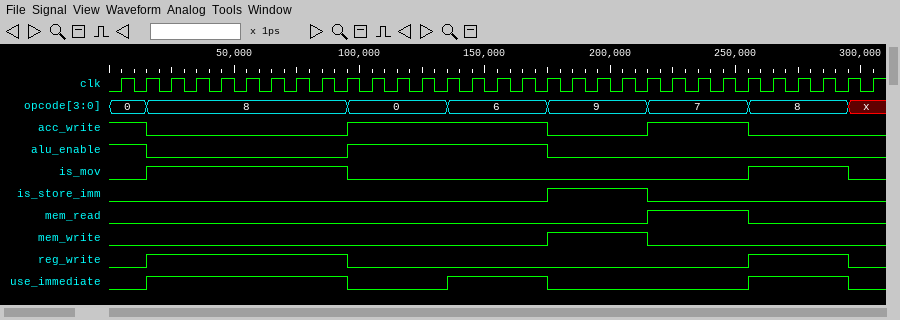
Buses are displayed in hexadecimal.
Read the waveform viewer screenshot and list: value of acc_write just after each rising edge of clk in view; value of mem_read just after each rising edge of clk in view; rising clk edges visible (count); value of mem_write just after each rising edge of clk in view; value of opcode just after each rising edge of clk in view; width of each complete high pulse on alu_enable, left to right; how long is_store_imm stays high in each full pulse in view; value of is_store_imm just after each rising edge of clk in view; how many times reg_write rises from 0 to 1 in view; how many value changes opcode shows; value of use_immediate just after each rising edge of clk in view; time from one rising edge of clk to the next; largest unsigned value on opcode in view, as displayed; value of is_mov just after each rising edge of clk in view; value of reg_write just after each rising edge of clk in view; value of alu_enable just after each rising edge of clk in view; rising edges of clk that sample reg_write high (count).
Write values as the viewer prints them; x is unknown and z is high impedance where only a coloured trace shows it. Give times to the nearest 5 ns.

1 0 0 0 0 0 0 0 0 1 1 1 1 1 1 1 1 0 0 0 0 1 1 1 1 0 0 0 0 0 0
0 0 0 0 0 0 0 0 0 0 0 0 0 0 0 0 0 0 0 0 0 1 1 1 1 0 0 0 0 0 0
31
0 0 0 0 0 0 0 0 0 0 0 0 0 0 0 0 0 1 1 1 1 0 0 0 0 0 0 0 0 0 0
0, 8, 8, 8, 8, 8, 8, 8, 8, 0, 0, 0, 0, 6, 6, 6, 6, 9, 9, 9, 9, 7, 7, 7, 7, 8, 8, 8, 8, x, x
80 ns
40 ns
0 0 0 0 0 0 0 0 0 0 0 0 0 0 0 0 0 1 1 1 1 0 0 0 0 0 0 0 0 0 0
2
7
0 1 1 1 1 1 1 1 1 0 0 0 0 1 1 1 1 0 0 0 0 0 0 0 0 1 1 1 1 0 0
10 ns
9
0 1 1 1 1 1 1 1 1 0 0 0 0 0 0 0 0 0 0 0 0 0 0 0 0 1 1 1 1 0 0
0 1 1 1 1 1 1 1 1 0 0 0 0 0 0 0 0 0 0 0 0 0 0 0 0 1 1 1 1 0 0
1 0 0 0 0 0 0 0 0 1 1 1 1 1 1 1 1 0 0 0 0 0 0 0 0 0 0 0 0 0 0
12
